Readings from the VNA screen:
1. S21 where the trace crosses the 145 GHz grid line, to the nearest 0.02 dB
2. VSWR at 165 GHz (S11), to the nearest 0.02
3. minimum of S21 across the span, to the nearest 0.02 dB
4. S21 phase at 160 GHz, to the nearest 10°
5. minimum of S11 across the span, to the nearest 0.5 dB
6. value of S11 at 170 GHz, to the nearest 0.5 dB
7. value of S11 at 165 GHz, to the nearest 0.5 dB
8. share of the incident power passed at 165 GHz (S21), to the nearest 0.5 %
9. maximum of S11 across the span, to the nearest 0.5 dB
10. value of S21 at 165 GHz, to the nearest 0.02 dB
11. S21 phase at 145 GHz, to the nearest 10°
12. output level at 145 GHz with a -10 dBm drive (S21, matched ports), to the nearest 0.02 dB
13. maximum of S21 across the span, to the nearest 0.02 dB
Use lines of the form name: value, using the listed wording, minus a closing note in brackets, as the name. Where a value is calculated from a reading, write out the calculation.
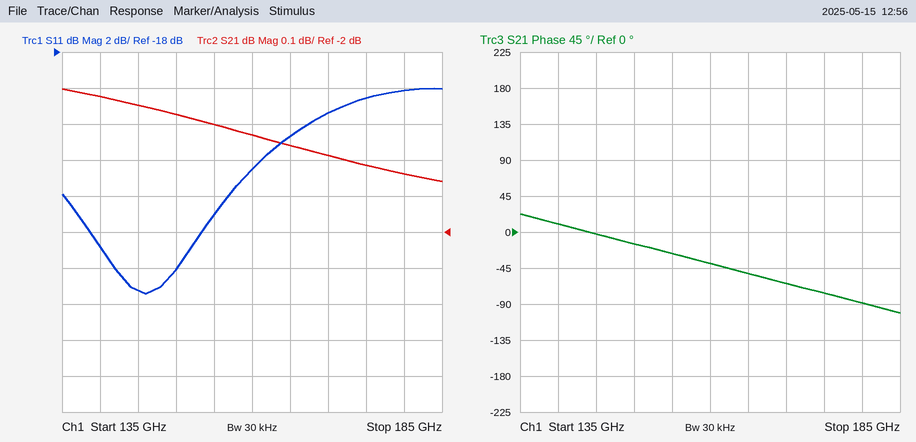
S21 where the trace crosses the 145 GHz grid line, to the nearest 0.02 dB: -1.64 dB
VSWR at 165 GHz (S11), to the nearest 0.02: |Γ| = 10^(-22.5/20) = 0.0750; VSWR = (1 + 0.0750)/(1 − 0.0750) ≈ 1.16
minimum of S21 across the span, to the nearest 0.02 dB: -1.86 dB
S21 phase at 160 GHz, to the nearest 10°: -40°
minimum of S11 across the span, to the nearest 0.5 dB: -31.5 dB
value of S11 at 170 GHz, to the nearest 0.5 dB: -21.5 dB
value of S11 at 165 GHz, to the nearest 0.5 dB: -22.5 dB
share of the incident power passed at 165 GHz (S21), to the nearest 0.5 %: 10^(-1.76/10) ≈ 66.7 %, so 66.5 % to the nearest 0.5 %
maximum of S11 across the span, to the nearest 0.5 dB: -20.0 dB
value of S21 at 165 GHz, to the nearest 0.02 dB: -1.76 dB
S21 phase at 145 GHz, to the nearest 10°: 0°
output level at 145 GHz with a -10 dBm drive (S21, matched ports), to the nearest 0.02 dB: -10 dBm + (-1.64 dB) = -11.64 dBm
maximum of S21 across the span, to the nearest 0.02 dB: -1.60 dB
